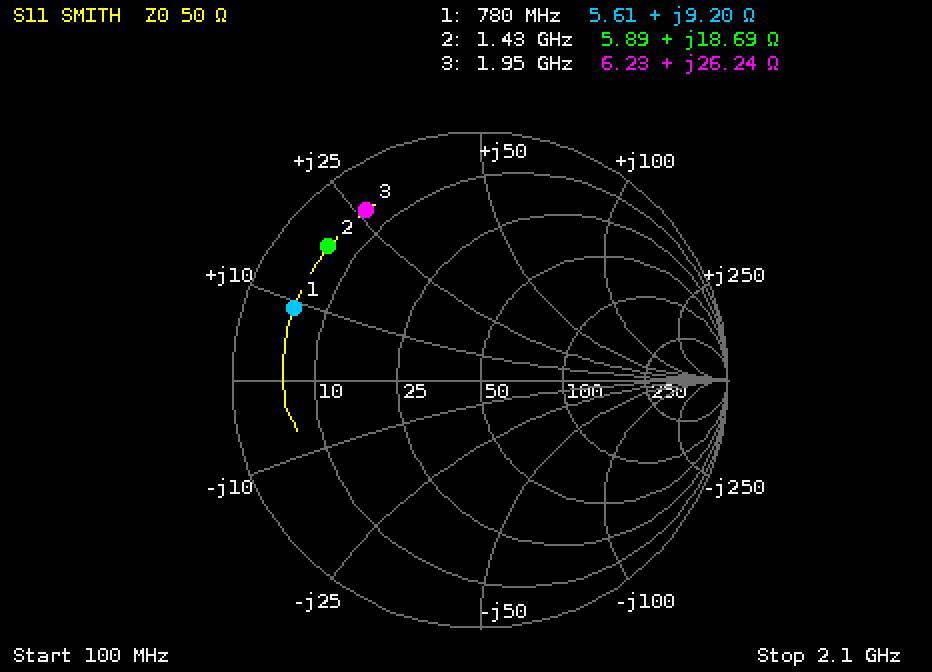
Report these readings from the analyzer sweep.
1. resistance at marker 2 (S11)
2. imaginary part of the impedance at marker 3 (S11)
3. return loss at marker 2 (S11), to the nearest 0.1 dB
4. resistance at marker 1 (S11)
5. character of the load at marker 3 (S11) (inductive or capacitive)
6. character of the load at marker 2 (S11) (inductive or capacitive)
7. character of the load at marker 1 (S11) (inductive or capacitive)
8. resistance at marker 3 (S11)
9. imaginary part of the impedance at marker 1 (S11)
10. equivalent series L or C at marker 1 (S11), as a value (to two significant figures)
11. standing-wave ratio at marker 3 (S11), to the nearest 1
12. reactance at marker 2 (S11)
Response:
5.89 Ω
+26.24 Ω
1.8 dB
5.61 Ω
inductive
inductive
inductive
6.23 Ω
+9.20 Ω
1.9 nH
10
+18.69 Ω
